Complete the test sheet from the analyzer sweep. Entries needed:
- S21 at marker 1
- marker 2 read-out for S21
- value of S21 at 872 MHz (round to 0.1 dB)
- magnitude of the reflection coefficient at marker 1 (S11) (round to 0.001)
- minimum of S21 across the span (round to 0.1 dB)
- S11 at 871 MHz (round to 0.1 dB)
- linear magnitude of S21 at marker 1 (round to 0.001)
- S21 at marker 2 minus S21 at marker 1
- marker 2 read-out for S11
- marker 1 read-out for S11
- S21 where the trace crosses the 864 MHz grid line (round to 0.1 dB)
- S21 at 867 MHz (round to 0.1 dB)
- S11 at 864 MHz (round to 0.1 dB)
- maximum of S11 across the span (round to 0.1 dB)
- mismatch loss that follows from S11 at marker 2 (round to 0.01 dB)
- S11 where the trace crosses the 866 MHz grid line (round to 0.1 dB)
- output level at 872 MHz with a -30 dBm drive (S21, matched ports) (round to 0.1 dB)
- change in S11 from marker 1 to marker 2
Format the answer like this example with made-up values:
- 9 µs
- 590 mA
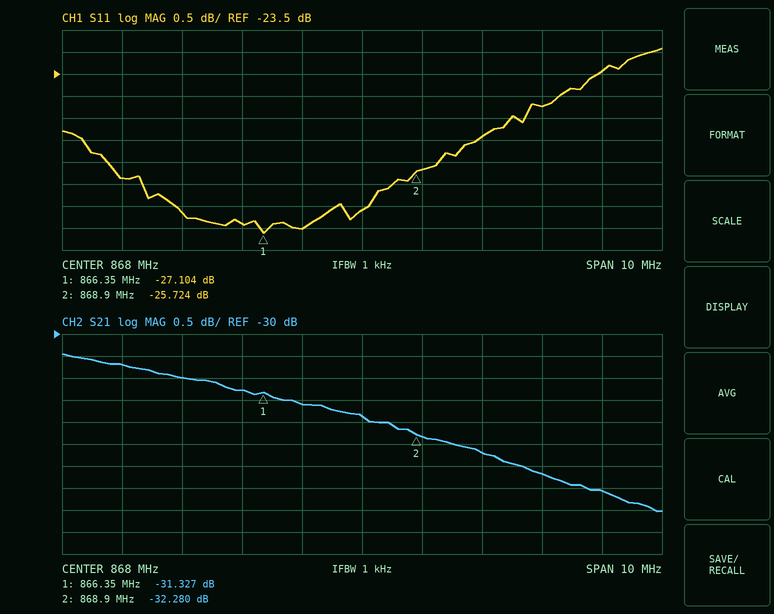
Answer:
- -31.327 dB
- -32.280 dB
- -33.6 dB
- 0.044
- -34.0 dB
- -24.2 dB
- 0.027
- -0.953 dB
- -25.724 dB
- -27.104 dB
- -30.7 dB
- -31.6 dB
- -25.9 dB
- -22.9 dB
- 0.01 dB
- -26.9 dB
- -63.6 dBm
- 1.380 dB
